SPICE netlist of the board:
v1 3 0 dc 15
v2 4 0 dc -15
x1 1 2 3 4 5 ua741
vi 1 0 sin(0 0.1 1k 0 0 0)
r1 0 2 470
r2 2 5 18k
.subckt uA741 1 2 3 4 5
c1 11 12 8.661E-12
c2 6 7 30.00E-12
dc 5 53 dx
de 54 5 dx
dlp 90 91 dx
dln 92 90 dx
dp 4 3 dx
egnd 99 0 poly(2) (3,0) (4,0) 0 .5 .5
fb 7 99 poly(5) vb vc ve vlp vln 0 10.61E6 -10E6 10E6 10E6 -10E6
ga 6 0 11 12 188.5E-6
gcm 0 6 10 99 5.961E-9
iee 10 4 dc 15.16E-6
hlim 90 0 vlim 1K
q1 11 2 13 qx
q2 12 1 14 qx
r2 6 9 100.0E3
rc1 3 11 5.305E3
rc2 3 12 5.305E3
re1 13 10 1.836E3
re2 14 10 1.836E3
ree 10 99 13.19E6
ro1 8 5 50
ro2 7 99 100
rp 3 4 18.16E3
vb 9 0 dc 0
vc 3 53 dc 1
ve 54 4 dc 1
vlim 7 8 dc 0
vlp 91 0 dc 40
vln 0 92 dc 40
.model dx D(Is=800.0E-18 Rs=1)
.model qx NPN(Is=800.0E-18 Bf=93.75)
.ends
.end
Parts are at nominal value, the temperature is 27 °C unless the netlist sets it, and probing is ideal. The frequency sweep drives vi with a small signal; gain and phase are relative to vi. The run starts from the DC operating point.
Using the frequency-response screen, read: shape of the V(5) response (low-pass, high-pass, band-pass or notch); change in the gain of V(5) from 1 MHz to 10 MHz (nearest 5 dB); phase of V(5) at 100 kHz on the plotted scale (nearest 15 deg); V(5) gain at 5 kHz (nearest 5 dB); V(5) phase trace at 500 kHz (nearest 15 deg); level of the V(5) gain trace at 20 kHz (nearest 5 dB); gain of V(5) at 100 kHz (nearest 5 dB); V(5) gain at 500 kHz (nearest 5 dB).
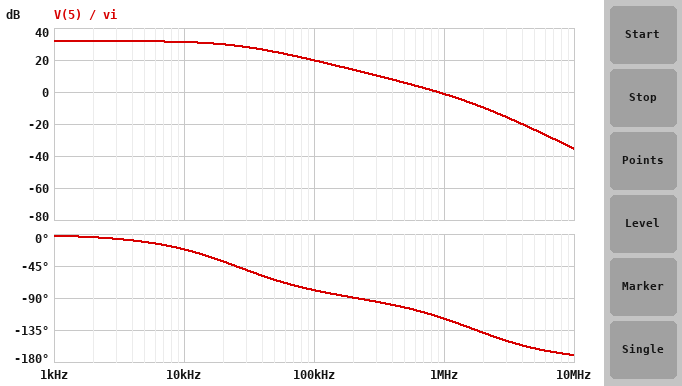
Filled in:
low-pass
-35 dB
-75 deg
30 dB
-105 deg
30 dB
20 dB
5 dB
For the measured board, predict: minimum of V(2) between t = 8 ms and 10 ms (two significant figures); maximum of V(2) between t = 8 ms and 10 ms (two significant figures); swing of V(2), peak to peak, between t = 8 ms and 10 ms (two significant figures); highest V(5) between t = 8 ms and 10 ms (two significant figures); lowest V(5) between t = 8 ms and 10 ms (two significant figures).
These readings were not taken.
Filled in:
-100 mV
100 mV
200 mV
3.9 V
-3.9 V
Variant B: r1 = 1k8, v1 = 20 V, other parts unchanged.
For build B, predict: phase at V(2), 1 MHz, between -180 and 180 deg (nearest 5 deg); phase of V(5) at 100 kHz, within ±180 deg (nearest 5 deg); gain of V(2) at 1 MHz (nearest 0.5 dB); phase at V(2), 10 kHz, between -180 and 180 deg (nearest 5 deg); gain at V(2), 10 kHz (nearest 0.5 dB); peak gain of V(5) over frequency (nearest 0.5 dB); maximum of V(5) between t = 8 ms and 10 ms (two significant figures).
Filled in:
-115 deg
-50 deg
-22.0 dB
-5 deg
0 dB
21.0 dB
1.1 V
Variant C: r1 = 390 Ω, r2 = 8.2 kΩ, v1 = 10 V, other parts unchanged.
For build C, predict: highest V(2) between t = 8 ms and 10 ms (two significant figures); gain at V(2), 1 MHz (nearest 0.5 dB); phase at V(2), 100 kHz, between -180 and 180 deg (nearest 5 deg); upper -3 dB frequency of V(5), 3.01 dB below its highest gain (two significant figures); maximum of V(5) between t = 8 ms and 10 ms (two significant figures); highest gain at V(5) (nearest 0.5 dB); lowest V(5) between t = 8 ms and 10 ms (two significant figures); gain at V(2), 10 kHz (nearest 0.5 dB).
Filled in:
100 mV
-28.0 dB
-70 deg
47 kHz
2.2 V
27.0 dB
-2.2 V
0 dB
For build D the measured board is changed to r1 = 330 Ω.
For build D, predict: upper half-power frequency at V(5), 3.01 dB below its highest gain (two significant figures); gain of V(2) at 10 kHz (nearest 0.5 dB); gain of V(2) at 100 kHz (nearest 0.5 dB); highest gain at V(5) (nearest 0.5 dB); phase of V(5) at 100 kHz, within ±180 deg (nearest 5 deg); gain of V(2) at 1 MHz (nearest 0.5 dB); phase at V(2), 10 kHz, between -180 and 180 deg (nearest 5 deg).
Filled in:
18 kHz
-1.0 dB
-15.0 dB
35.0 dB
-85 deg
-36.0 dB
-30 deg
